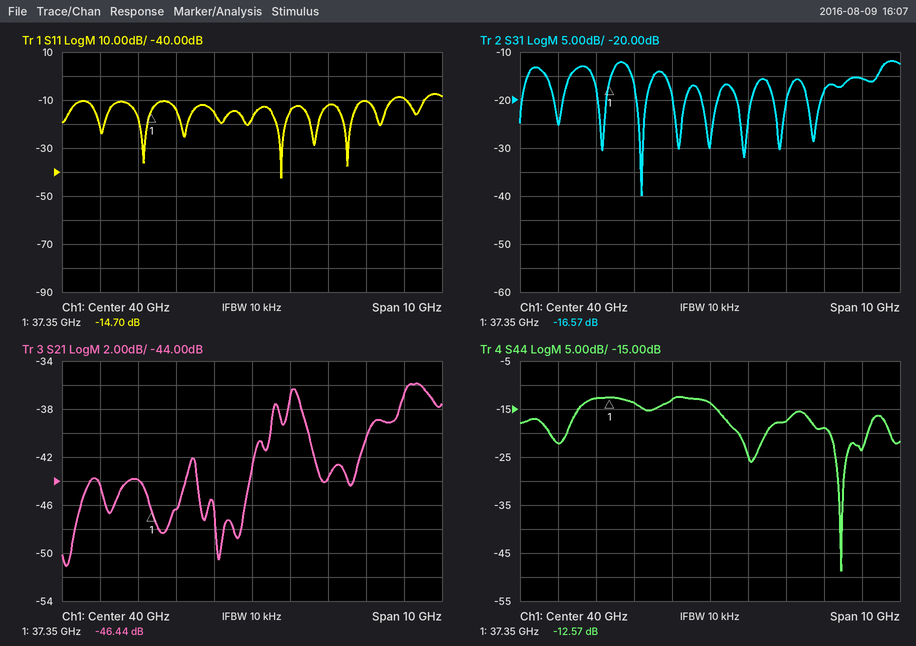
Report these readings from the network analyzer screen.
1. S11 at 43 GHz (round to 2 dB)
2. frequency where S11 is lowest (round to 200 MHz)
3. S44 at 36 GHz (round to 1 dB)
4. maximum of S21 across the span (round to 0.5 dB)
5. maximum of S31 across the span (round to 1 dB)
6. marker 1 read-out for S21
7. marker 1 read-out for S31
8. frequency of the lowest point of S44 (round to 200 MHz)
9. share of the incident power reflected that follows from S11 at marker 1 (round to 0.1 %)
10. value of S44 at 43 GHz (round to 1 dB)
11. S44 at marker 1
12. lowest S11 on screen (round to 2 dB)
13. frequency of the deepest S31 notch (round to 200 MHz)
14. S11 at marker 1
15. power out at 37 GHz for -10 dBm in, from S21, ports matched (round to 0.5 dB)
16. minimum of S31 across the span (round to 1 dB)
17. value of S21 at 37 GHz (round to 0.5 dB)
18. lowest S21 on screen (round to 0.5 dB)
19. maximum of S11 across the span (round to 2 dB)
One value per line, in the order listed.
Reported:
-10 dB
40.8 GHz
-22 dB
-36.0 dB
-12 dB
-46.44 dB
-16.57 dB
43.4 GHz
3.4 %
-19 dB
-12.57 dB
-42 dB
38.2 GHz
-14.70 dB
-54.0 dBm
-40 dB
-44.0 dB
-51.0 dB
-8 dB
